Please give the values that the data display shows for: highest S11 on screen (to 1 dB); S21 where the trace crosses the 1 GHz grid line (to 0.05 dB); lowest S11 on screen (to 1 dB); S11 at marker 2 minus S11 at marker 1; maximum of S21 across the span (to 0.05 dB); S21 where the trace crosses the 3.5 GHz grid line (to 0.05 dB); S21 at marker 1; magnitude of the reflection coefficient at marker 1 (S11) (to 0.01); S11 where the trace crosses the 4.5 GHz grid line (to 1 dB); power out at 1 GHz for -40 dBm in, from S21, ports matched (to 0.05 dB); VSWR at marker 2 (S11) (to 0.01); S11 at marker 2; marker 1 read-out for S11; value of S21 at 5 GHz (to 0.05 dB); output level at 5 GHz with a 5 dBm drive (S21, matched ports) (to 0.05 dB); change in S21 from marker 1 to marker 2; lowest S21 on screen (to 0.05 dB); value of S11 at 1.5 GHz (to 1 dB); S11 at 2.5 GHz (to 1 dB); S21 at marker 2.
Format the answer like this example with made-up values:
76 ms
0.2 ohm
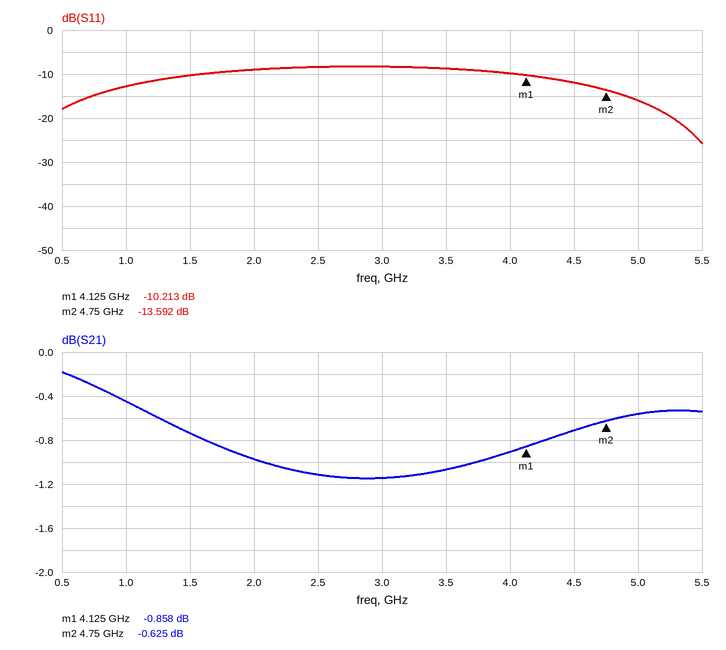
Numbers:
-8 dB
-0.45 dB
-26 dB
-3.379 dB
-0.20 dB
-1.05 dB
-0.858 dB
0.31
-12 dB
-40.45 dBm
1.53
-13.592 dB
-10.213 dB
-0.55 dB
4.45 dBm
0.233 dB
-1.15 dB
-10 dB
-8 dB
-0.625 dB
